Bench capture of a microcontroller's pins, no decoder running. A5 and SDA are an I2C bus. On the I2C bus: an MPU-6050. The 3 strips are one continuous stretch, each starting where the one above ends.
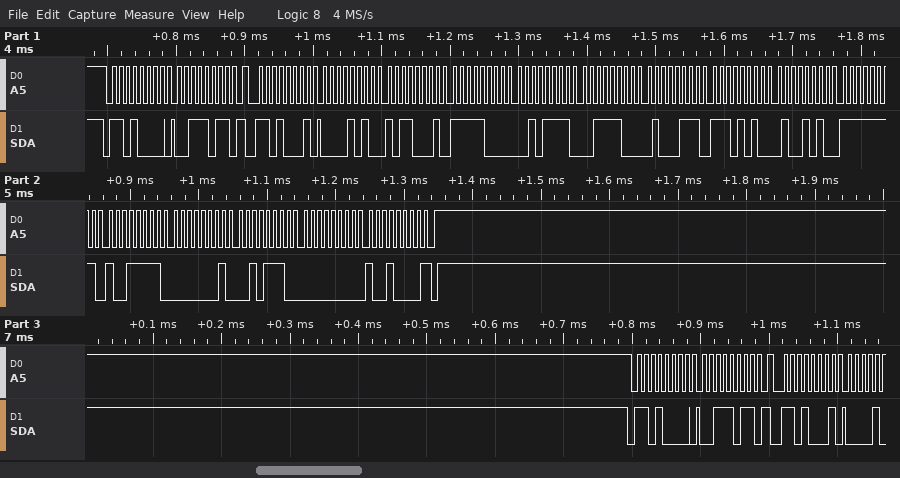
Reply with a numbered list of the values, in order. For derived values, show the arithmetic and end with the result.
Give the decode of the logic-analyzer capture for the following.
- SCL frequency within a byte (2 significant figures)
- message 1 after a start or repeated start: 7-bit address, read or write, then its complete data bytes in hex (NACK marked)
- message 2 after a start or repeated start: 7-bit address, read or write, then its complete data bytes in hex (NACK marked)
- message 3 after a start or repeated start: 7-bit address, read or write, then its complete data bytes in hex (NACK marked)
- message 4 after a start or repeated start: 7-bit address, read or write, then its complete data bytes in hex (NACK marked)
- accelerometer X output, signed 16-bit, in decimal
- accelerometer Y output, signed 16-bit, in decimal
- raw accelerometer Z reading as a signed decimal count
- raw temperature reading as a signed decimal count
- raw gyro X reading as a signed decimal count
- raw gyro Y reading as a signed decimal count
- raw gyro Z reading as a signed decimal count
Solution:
1. 100 kHz
2. 0x68 write: 3B
3. 0x68 read: 0A B1 F8 2F 3C 47 EA 4A FF 9F 01 2E 00 90 NACK
4. 0x68 write: 3B
5. 0x68 read
6. 0x0AB1 = 2737
7. 0xF82F = -2001
8. 0x3C47 = 15431
9. 0xEA4A = -5558
10. 0xFF9F = -97
11. 0x012E = 302
12. 0x0090 = 144
